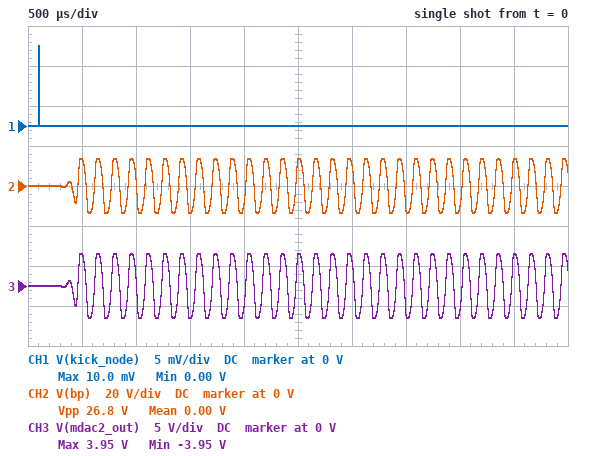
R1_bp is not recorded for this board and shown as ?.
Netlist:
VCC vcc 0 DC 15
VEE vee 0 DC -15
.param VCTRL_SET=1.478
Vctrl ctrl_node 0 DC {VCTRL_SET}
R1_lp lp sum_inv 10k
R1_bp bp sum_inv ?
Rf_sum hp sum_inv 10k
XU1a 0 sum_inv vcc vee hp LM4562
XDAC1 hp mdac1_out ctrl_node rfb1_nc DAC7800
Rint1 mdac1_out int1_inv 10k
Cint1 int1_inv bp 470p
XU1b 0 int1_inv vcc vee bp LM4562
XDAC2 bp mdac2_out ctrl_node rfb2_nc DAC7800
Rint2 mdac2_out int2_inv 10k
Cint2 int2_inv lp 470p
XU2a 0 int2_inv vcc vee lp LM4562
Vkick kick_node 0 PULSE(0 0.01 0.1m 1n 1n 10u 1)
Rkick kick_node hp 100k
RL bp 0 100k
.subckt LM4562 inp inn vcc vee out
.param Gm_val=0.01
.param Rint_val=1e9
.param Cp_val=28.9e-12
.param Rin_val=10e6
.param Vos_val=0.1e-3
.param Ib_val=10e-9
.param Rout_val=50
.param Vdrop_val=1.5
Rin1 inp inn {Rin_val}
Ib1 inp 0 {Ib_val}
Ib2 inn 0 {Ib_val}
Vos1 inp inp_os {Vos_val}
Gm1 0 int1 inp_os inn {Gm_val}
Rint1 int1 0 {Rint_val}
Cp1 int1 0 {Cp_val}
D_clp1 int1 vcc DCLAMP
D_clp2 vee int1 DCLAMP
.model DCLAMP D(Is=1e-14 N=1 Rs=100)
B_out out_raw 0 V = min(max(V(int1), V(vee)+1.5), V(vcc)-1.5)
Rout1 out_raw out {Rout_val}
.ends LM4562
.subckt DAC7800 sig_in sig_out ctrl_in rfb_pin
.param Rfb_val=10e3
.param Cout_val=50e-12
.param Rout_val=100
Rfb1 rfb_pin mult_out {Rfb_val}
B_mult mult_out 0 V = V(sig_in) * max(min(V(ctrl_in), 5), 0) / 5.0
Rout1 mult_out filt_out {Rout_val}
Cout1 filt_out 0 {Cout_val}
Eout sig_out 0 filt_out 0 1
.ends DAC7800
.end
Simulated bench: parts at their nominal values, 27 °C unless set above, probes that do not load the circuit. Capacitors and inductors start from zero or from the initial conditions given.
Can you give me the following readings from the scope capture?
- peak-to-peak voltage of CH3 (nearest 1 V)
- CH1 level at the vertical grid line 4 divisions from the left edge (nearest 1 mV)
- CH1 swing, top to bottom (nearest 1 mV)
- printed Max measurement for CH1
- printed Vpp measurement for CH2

8 V
0 V
10 mV
10.0 mV
26.8 V
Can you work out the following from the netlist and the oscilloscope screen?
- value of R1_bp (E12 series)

12 kΩ
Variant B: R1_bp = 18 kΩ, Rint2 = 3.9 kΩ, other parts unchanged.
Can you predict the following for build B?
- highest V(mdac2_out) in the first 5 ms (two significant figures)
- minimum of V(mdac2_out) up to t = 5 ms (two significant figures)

3.4 V
-3.4 V
